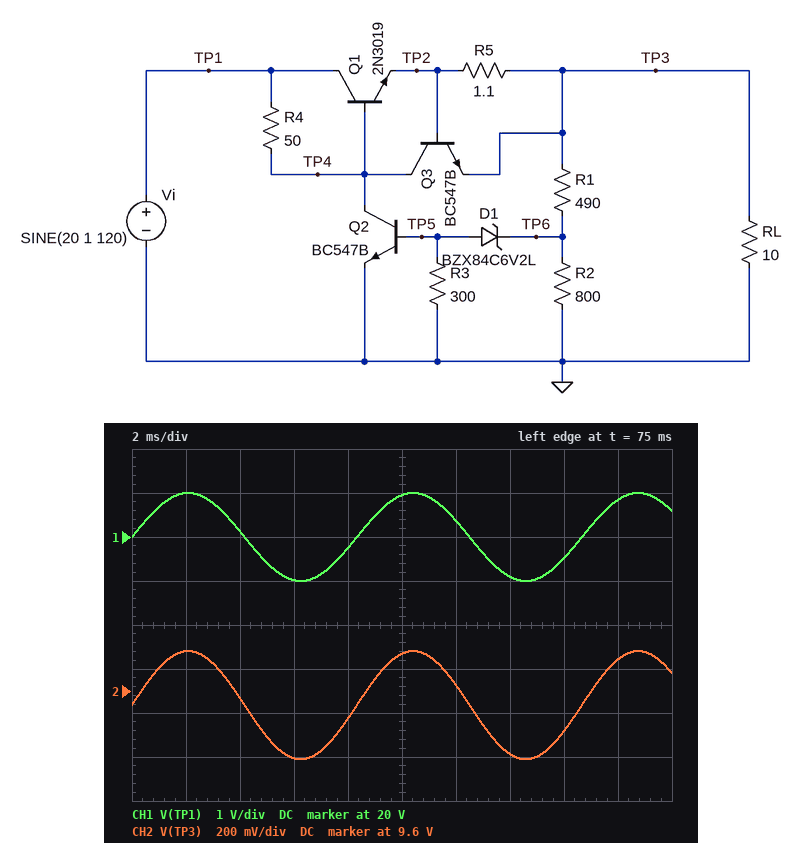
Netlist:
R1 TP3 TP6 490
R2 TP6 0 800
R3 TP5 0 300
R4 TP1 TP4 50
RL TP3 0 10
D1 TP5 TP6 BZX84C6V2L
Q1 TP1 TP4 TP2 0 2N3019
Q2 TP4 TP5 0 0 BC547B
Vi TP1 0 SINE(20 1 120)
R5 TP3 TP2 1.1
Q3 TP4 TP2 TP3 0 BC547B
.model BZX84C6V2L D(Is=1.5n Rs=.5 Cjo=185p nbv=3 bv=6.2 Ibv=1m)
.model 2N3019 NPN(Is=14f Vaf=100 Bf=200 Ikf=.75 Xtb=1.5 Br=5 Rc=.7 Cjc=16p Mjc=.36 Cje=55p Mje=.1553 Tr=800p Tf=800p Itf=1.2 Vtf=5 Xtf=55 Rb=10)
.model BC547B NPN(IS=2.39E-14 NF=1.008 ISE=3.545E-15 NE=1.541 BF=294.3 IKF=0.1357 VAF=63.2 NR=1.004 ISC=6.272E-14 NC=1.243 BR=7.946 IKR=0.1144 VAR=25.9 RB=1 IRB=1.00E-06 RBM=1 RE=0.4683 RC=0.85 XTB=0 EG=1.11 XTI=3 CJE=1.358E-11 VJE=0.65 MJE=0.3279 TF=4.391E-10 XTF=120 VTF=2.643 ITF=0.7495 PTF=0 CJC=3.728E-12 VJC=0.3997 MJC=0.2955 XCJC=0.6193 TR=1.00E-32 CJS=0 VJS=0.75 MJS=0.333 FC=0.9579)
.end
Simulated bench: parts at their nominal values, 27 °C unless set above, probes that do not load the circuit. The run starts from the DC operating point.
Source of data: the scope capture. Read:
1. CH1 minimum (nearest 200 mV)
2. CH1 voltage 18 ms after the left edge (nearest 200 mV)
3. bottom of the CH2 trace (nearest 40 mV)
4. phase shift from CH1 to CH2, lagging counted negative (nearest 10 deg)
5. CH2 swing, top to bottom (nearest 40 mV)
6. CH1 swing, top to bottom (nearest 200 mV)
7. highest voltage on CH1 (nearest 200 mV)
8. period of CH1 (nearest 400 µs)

19.0 V
20.8 V
9.28 V
0 deg
480 mV
2.0 V
21.0 V
8.4 ms
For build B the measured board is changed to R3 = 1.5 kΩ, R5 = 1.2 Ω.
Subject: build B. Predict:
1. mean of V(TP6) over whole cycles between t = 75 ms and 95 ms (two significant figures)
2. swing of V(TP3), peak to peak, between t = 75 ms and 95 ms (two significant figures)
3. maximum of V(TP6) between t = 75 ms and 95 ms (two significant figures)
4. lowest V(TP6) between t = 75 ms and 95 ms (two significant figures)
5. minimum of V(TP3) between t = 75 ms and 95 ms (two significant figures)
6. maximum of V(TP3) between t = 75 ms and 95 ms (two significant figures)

5.6 V
480 mV
5.8 V
5.5 V
8.8 V
9.3 V
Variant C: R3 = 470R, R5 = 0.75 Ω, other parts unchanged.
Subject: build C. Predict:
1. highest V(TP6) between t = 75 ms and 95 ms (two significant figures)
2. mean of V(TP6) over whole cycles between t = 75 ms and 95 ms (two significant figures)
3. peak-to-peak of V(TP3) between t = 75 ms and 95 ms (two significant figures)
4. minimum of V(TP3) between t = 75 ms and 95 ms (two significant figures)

7.0 V
6.9 V
280 mV
12 V
